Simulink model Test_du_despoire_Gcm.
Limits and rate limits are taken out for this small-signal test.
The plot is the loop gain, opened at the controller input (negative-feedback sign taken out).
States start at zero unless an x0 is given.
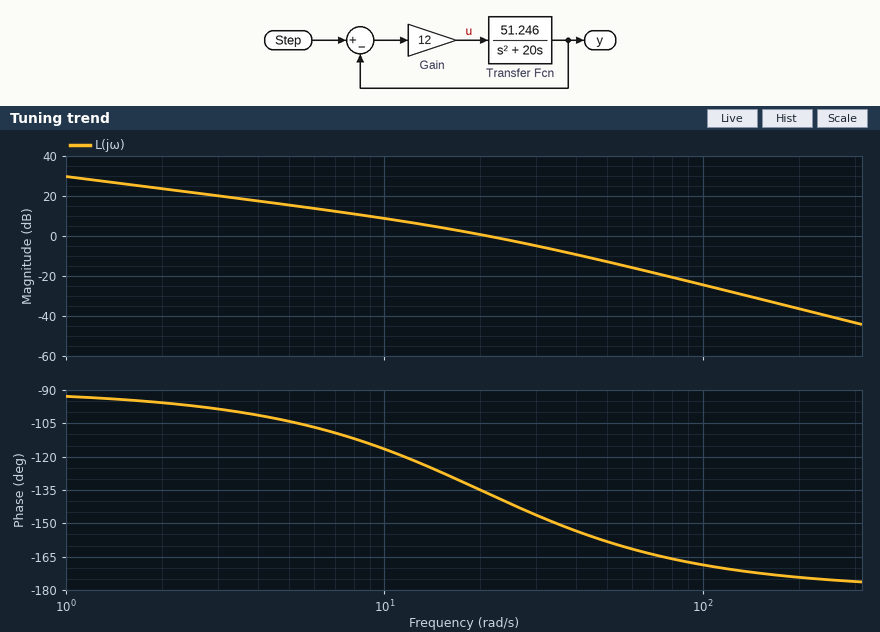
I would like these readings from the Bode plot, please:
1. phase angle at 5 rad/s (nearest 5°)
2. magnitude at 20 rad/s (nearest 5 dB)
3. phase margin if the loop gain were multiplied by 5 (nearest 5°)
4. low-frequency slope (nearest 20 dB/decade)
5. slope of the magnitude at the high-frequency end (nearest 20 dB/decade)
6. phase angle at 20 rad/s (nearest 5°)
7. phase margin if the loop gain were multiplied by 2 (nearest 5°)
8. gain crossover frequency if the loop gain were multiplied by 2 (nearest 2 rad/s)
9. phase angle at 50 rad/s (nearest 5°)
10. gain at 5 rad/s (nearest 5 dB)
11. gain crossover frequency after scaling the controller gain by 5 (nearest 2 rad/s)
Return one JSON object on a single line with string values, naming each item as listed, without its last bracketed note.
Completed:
{"phase angle at 5 rad/s": "-105°", "magnitude at 20 rad/s": "0 dB", "phase margin if the loop gain were multiplied by 5": "20°", "low-frequency slope": "-20 dB/decade", "slope of the magnitude at the high-frequency end": "-40 dB/decade", "phase angle at 20 rad/s": "-135°", "phase margin if the loop gain were multiplied by 2": "30°", "gain crossover frequency if the loop gain were multiplied by 2": "32 rad/s", "phase angle at 50 rad/s": "-160°", "gain at 5 rad/s": "15 dB", "gain crossover frequency after scaling the controller gain by 5": "54 rad/s"}
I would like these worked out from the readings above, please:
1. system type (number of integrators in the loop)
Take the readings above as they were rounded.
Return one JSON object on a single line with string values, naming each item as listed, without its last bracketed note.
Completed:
{"system type": "1"}
